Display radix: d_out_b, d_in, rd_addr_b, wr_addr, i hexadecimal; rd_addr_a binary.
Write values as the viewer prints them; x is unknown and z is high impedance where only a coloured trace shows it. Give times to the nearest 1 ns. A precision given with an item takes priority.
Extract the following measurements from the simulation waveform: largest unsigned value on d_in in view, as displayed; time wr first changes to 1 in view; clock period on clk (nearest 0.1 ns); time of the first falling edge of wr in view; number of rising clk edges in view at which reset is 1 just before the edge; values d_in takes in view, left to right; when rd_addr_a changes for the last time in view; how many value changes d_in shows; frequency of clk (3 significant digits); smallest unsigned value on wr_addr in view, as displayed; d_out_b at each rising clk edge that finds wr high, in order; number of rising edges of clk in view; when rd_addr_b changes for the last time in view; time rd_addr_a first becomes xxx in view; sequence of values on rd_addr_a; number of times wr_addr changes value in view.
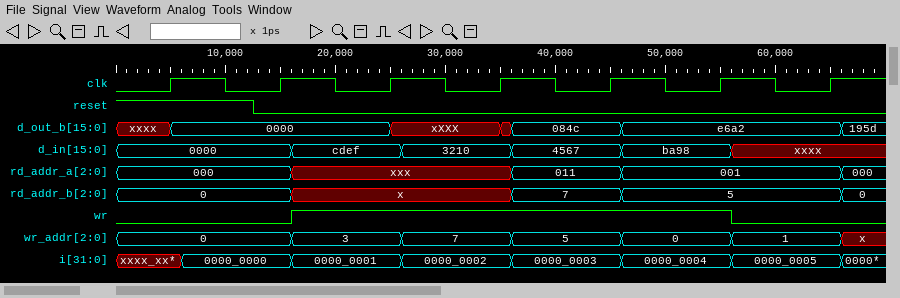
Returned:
cdef
16 ns
10 ns
56 ns
1
0000, cdef, 3210, 4567, ba98, xxxx
66 ns
5
100 MHz
0
0000, xXXX, 084c, e6a2
7
66 ns
16 ns
000, xxx, 011, 001, 000
6
